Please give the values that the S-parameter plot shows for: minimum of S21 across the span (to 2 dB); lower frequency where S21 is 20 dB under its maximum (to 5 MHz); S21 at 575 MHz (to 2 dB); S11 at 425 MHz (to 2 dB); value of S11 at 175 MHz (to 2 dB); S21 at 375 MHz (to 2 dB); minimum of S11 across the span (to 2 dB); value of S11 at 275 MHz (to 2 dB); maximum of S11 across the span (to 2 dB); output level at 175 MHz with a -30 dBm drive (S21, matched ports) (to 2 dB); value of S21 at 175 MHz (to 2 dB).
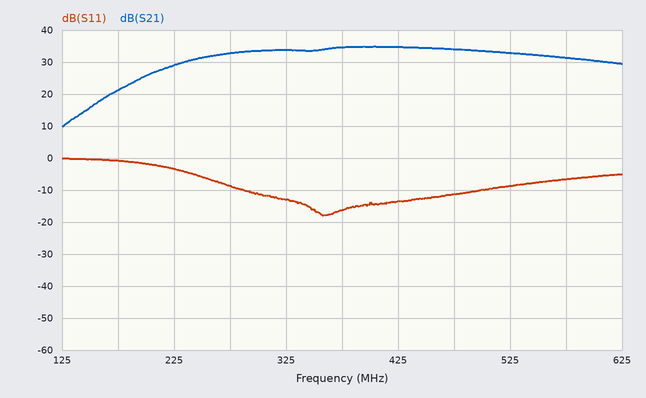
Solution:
10 dB
145 MHz
32 dB
-14 dB
0 dB
34 dB
-18 dB
-8 dB
0 dB
-8 dBm
22 dB
